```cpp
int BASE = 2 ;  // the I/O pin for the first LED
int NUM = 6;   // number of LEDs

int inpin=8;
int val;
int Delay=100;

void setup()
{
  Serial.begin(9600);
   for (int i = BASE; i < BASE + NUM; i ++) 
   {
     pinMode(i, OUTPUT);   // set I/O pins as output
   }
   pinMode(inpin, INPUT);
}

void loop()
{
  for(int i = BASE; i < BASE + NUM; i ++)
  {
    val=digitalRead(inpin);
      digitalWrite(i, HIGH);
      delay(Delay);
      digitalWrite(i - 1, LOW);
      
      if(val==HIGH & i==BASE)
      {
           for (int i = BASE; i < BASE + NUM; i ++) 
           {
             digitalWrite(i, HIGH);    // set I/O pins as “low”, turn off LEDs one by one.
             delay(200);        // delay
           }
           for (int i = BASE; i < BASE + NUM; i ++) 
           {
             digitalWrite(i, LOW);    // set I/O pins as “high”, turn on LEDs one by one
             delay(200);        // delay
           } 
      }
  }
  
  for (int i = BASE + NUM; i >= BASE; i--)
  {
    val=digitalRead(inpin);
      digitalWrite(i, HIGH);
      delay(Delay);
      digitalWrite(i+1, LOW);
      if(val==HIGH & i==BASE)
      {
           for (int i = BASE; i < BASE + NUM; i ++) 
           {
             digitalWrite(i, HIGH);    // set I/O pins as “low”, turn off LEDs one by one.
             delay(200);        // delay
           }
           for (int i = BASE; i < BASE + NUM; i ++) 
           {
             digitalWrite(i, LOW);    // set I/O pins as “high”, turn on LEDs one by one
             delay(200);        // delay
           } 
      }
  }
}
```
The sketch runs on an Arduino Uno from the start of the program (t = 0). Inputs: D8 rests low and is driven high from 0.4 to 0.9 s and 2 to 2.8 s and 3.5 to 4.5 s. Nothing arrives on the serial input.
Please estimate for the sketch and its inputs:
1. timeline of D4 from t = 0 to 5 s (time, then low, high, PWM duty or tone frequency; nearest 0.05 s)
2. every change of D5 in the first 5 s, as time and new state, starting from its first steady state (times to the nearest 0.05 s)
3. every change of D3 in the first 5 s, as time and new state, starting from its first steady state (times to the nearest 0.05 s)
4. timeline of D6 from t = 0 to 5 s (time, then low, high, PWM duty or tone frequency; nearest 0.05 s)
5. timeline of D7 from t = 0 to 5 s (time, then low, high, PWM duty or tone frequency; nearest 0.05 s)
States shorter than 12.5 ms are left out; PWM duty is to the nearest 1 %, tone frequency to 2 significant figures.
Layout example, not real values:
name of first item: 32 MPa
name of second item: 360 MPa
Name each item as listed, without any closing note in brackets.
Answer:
timeline of D4 from t = 0 to 5 s: 0 s low; 0.2 s high; 0.4 s low; 1 s high; 1.2 s low; 1.5 s high; 1.7 s low; 2.3 s high; 2.5 s low; 3 s high; 4.2 s low
every change of D5 in the first 5 s, as time and new state, starting from its first steady state: 0 s low; 0.3 s high; 0.5 s low; 0.9 s high; 1.1 s low; 1.6 s high; 1.8 s low; 2.2 s high; 2.4 s low; 3.2 s high; 4.4 s low
every change of D3 in the first 5 s, as time and new state, starting from its first steady state: 0 s low; 0.1 s high; 0.3 s low; 1.1 s high; 1.3 s low; 1.4 s high; 1.6 s low; 2.4 s high; 2.6 s low; 2.8 s high; 4 s low
timeline of D6 from t = 0 to 5 s: 0 s low; 0.4 s high; 0.6 s low; 0.8 s high; 1 s low; 1.7 s high; 1.9 s low; 2.1 s high; 2.3 s low; 3.4 s high; 4.6 s low
timeline of D7 from t = 0 to 5 s: 0 s low; 0.5 s high; 0.9 s low; 1.8 s high; 2.2 s low; 3.6 s high; 4.8 s low
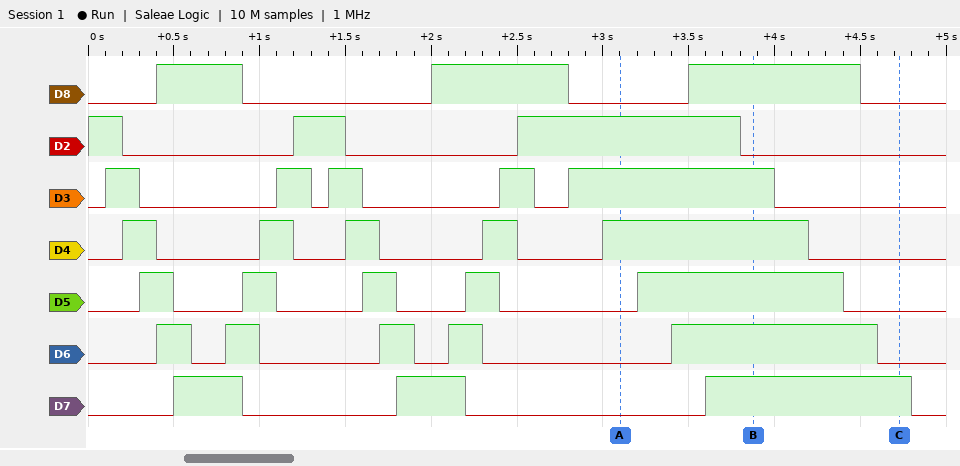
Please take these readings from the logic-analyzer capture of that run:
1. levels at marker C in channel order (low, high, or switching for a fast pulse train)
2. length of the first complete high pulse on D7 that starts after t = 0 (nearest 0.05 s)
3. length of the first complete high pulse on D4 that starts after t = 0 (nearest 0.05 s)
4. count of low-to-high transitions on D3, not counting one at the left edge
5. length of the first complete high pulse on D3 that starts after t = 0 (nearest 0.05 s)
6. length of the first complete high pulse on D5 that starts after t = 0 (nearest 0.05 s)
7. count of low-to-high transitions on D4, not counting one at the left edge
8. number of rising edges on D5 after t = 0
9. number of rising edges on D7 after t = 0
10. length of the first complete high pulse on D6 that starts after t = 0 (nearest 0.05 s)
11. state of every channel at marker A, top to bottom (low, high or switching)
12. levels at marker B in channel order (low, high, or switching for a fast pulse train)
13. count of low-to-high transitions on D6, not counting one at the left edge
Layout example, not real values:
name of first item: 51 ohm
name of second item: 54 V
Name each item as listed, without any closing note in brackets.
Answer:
levels at marker C in channel order: D8 low, D2 low, D3 low, D4 low, D5 low, D6 low, D7 high
length of the first complete high pulse on D7 that starts after t = 0: 0.40 s
length of the first complete high pulse on D4 that starts after t = 0: 0.20 s
count of low-to-high transitions on D3, not counting one at the left edge: 5
length of the first complete high pulse on D3 that starts after t = 0: 0.20 s
length of the first complete high pulse on D5 that starts after t = 0: 0.20 s
count of low-to-high transitions on D4, not counting one at the left edge: 5
number of rising edges on D5 after t = 0: 5
number of rising edges on D7 after t = 0: 3
length of the first complete high pulse on D6 that starts after t = 0: 0.20 s
state of every channel at marker A, top to bottom: D8 low, D2 high, D3 high, D4 high, D5 low, D6 low, D7 low
levels at marker B in channel order: D8 high, D2 low, D3 high, D4 high, D5 high, D6 high, D7 high
count of low-to-high transitions on D6, not counting one at the left edge: 5
